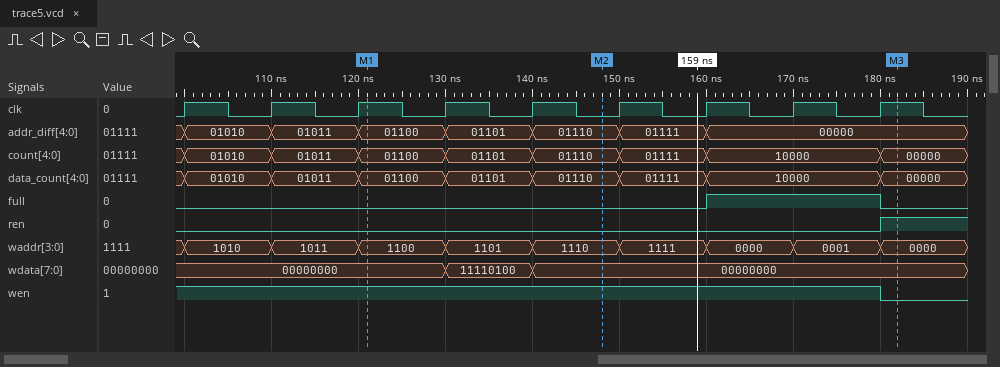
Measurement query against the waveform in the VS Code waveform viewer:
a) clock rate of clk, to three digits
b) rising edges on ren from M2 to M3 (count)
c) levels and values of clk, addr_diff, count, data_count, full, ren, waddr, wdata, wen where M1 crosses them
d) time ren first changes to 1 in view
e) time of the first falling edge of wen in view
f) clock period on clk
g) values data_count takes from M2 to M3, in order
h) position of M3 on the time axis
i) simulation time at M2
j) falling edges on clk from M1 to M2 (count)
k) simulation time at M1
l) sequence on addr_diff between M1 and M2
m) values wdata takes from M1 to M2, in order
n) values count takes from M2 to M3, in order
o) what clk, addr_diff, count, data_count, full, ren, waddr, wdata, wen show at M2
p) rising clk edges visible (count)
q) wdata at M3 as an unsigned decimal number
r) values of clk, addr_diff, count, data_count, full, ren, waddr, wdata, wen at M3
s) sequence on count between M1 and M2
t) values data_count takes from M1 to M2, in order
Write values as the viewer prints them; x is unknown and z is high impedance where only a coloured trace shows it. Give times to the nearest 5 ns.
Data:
100 MHz
1
clk=1, addr_diff=01100, count=01100, data_count=01100, full=0, ren=0, waddr=1100, wdata=00000000, wen=1
180 ns
180 ns
10 ns
01110, 01111, 10000, 00000
180 ns
150 ns
3
120 ns
01100, 01101, 01110
00000000, 11110100, 00000000
01110, 01111, 10000, 00000
clk=0, addr_diff=01110, count=01110, data_count=01110, full=0, ren=0, waddr=1110, wdata=00000000, wen=1
9
0
clk=1, addr_diff=00000, count=00000, data_count=00000, full=0, ren=1, waddr=0000, wdata=00000000, wen=0
01100, 01101, 01110
01100, 01101, 01110
